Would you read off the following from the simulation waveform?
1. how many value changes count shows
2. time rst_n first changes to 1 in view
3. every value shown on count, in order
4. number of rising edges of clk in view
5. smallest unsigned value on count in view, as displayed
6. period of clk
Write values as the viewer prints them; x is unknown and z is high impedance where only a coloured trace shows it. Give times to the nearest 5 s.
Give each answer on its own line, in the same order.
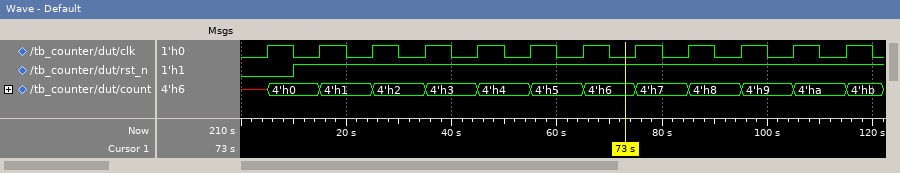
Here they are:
12
10 s
x, 4'h0, 4'h1, 4'h2, 4'h3, 4'h4, 4'h5, 4'h6, 4'h7, 4'h8, 4'h9, 4'ha, 4'hb
12
4'h0
10 s
